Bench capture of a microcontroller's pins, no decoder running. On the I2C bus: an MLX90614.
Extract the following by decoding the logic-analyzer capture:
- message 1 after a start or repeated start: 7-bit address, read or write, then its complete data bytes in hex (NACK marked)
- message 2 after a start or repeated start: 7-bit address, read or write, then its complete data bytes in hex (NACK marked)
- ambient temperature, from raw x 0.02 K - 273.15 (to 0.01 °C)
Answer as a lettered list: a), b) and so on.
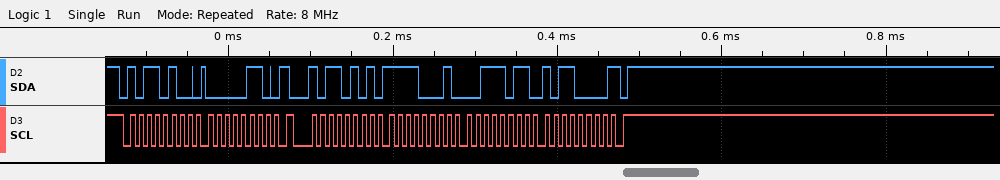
a) 0x5A write: 06
b) 0x5A read: F1 3B B0 NACK
c) 33.75 °C
